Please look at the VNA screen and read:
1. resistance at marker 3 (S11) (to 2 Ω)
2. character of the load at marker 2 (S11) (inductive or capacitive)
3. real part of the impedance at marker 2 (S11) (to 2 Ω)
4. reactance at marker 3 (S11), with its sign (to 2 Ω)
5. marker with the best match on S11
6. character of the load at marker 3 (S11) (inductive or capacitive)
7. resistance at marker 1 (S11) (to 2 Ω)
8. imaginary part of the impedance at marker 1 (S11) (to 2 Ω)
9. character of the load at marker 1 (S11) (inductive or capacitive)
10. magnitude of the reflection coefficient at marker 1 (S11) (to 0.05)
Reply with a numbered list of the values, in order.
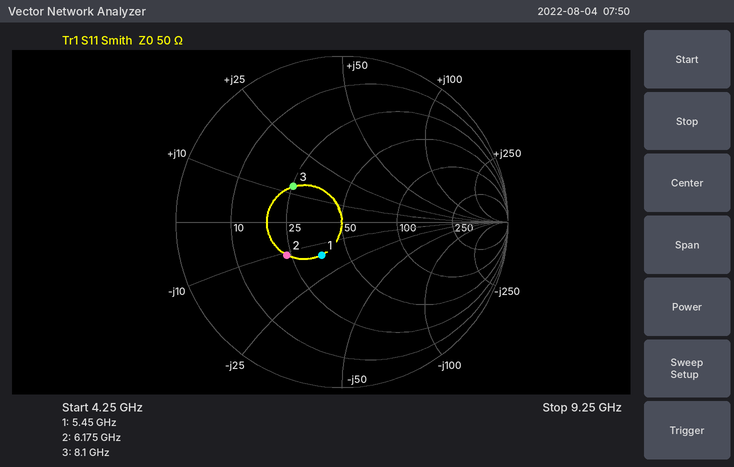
1. 26 Ω
2. capacitive
3. 24 Ω
4. +12 Ω
5. marker 1
6. inductive
7. 36 Ω
8. -16 Ω
9. capacitive
10. 0.25
